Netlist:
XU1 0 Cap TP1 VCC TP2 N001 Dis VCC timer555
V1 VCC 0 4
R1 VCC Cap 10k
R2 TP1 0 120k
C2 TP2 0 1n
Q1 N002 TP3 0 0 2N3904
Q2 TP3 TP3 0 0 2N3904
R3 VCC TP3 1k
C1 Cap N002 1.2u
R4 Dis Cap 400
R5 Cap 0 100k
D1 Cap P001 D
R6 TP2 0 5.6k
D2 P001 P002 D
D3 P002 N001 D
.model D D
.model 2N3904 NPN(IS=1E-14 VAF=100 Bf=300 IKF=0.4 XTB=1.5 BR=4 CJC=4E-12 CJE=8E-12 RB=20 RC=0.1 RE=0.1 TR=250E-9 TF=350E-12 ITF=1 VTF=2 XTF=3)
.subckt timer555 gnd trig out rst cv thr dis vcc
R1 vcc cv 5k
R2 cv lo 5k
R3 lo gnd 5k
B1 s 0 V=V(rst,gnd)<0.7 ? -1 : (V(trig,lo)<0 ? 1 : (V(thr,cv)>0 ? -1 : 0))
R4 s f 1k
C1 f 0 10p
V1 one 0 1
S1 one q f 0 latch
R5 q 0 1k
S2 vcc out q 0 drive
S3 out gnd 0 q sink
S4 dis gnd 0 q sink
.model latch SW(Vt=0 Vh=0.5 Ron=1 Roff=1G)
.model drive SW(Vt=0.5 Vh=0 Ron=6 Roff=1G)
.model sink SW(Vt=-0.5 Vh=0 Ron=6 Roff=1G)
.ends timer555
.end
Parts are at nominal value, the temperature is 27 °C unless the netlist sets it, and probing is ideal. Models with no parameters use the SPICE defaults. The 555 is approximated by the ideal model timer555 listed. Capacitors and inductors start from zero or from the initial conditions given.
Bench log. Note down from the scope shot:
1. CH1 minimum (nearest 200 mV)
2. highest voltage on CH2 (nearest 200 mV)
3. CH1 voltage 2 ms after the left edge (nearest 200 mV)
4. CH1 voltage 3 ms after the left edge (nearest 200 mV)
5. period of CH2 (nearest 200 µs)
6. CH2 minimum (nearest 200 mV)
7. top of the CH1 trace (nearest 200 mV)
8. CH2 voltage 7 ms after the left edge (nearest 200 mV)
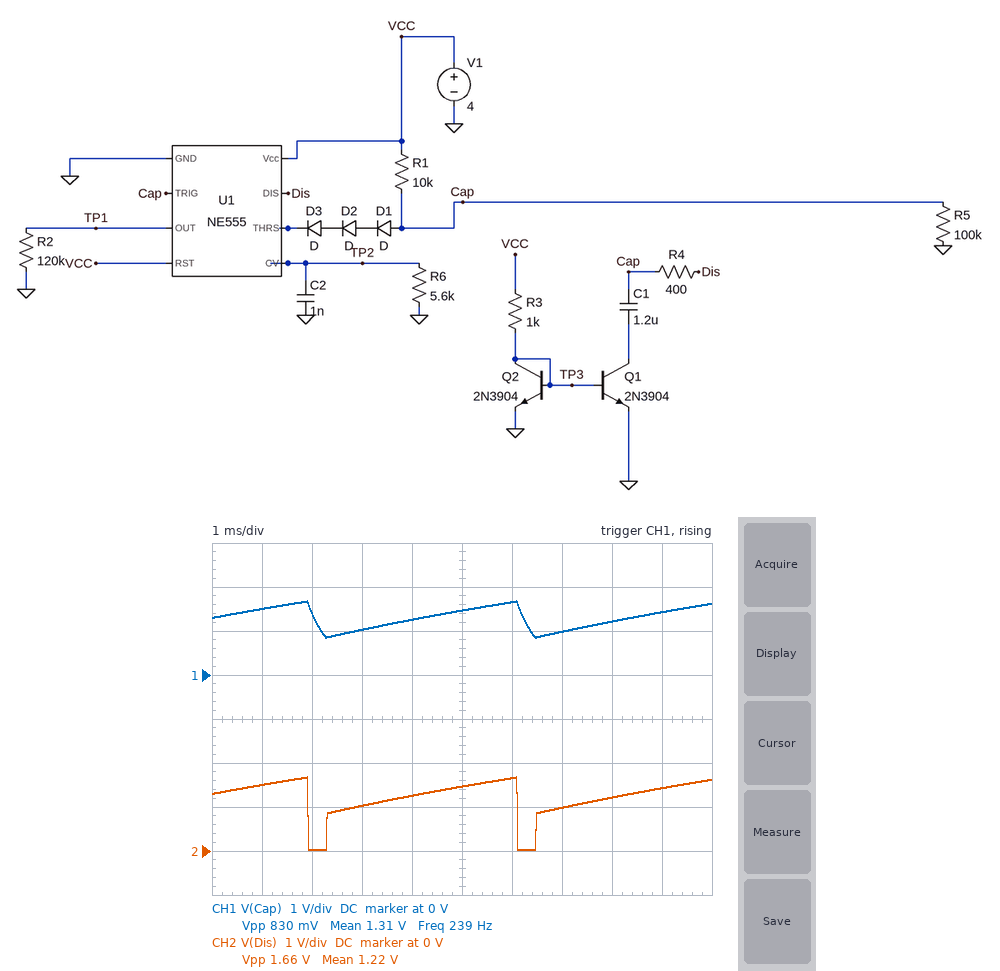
800 mV
1.6 V
1.4 V
1.0 V
4.2 ms
0 V
1.6 V
1.0 V
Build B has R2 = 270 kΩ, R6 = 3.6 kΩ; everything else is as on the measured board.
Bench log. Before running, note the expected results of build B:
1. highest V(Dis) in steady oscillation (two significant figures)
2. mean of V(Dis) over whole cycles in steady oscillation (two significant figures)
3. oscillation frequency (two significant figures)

1.4 V
940 mV
310 Hz
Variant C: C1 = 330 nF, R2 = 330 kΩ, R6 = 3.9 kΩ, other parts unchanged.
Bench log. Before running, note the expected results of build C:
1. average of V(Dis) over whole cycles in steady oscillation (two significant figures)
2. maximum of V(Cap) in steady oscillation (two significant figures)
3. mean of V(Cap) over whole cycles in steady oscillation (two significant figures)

980 mV
1.4 V
1.1 V
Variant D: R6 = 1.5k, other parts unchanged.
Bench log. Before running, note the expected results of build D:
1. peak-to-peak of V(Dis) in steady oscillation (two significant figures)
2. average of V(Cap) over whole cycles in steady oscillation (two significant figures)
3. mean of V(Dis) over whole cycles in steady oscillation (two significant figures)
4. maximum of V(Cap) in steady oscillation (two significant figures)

820 mV
620 mV
490 mV
830 mV
